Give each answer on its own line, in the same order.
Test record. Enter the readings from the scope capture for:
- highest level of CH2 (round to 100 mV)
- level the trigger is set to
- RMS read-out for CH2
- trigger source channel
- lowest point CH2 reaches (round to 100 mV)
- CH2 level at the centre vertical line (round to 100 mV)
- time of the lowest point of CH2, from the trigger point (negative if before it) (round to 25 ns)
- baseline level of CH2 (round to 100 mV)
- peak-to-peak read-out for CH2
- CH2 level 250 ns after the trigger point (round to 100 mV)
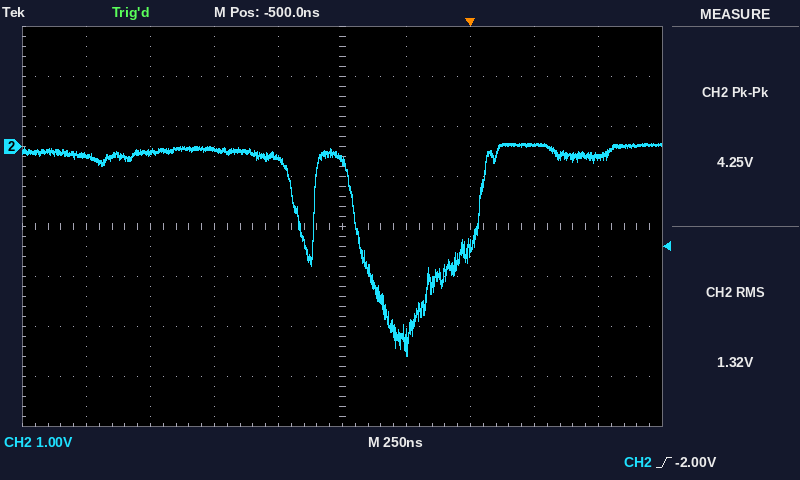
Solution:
100 mV
-2.00 V
1.32 V
CH2
-4.2 V
-300 mV
-250 ns
-100 mV
4.25 V
0.0 V
